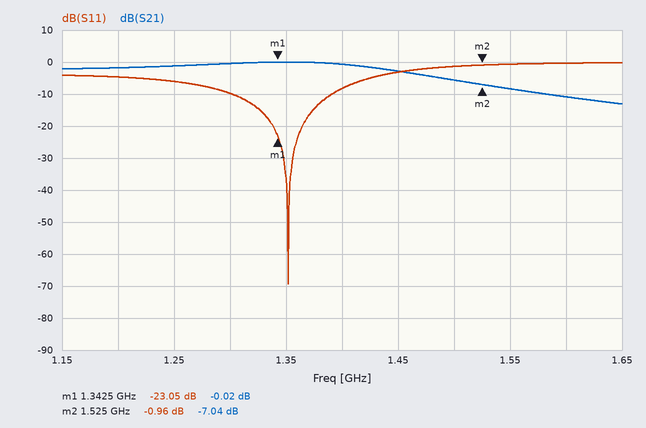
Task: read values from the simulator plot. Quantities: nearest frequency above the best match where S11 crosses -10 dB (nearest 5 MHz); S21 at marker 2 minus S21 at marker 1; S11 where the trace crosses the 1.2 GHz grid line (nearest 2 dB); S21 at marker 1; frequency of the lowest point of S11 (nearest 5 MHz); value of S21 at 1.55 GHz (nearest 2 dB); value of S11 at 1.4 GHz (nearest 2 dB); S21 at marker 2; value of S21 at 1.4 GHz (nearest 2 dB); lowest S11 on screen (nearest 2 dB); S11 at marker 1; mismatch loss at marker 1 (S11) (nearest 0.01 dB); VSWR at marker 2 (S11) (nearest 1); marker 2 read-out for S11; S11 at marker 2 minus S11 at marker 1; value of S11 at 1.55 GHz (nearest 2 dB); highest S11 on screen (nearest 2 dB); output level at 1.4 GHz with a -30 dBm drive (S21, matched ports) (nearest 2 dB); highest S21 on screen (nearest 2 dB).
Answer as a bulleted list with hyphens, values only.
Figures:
- 1.390 GHz
- -7.02 dB
- -4 dB
- -0.02 dB
- 1.350 GHz
- -8 dB
- -8 dB
- -7.04 dB
- 0 dB
- -70 dB
- -23.05 dB
- 0.02 dB
- 18
- -0.96 dB
- 22.09 dB
- 0 dB
- 0 dB
- -30 dBm
- 0 dB
